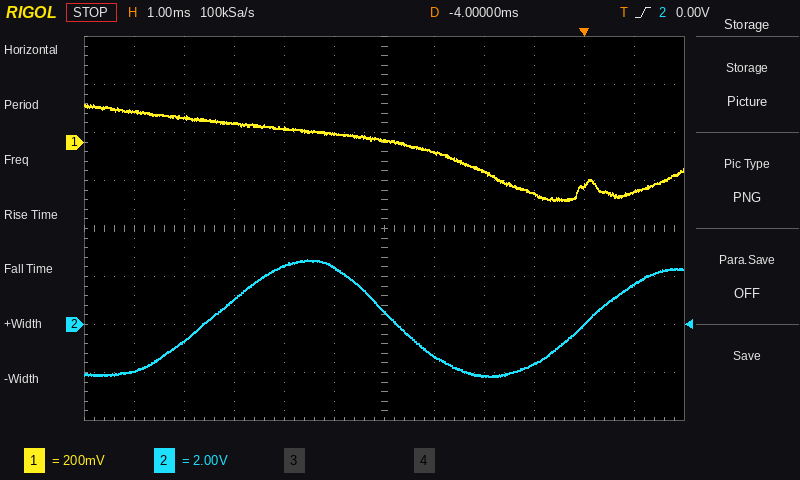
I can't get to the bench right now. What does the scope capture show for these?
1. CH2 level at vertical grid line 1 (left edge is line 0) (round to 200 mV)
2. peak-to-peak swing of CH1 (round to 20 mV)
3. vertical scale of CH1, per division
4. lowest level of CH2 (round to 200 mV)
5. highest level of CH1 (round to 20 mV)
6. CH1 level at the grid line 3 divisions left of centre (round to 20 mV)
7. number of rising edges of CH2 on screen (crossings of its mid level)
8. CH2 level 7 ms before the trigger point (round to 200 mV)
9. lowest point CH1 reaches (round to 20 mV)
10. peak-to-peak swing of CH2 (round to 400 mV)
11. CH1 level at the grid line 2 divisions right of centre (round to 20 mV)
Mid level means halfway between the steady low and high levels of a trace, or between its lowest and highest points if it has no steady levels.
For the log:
-2.0 V
400 mV
200 mV
-2.2 V
160 mV
80 mV
2
1.0 V
-240 mV
4.8 V
-120 mV
